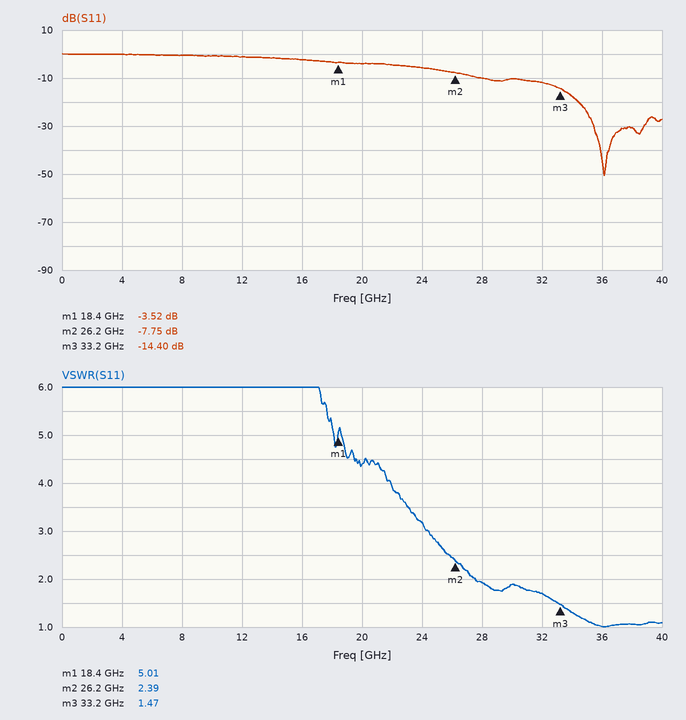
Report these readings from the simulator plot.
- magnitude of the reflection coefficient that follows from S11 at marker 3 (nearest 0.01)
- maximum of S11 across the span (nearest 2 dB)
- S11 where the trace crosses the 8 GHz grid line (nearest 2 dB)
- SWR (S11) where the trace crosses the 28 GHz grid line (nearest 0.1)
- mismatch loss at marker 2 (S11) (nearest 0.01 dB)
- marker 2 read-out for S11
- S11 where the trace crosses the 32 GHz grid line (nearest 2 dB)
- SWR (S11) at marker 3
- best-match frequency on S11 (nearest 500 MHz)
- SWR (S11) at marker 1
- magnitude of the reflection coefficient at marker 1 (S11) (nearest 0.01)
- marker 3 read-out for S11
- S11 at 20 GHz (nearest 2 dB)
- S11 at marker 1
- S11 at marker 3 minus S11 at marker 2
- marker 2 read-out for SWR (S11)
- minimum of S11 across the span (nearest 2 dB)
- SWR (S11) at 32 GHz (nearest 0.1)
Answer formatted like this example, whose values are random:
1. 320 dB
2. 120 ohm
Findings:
1. 0.19
2. 0 dB
3. 0 dB
4. 1.9
5. 0.80 dB
6. -7.75 dB
7. -12 dB
8. 1.47
9. 36.0 GHz
10. 5.01
11. 0.67
12. -14.40 dB
13. -4 dB
14. -3.52 dB
15. -6.65 dB
16. 2.39
17. -50 dB
18. 1.7
